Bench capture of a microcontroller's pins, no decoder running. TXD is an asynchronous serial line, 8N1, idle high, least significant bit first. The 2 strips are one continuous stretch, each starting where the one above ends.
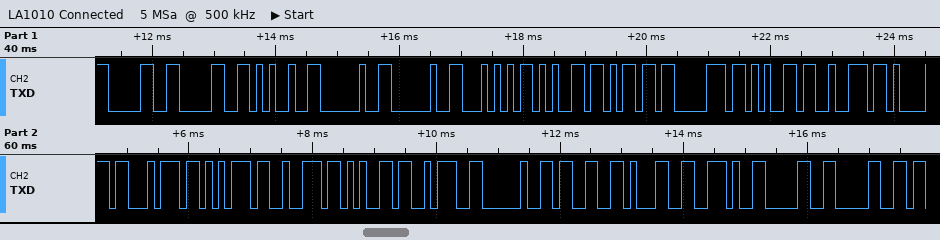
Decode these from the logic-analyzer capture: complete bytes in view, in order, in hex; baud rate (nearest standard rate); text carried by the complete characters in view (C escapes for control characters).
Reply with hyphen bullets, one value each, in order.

- 30 30 25 20 20 54 65 6D 70 65 72 61 74 75 72 65 3A 20 33 31 2E 30 30
- 9600 baud
- "00%  Temperature: 31.00"
